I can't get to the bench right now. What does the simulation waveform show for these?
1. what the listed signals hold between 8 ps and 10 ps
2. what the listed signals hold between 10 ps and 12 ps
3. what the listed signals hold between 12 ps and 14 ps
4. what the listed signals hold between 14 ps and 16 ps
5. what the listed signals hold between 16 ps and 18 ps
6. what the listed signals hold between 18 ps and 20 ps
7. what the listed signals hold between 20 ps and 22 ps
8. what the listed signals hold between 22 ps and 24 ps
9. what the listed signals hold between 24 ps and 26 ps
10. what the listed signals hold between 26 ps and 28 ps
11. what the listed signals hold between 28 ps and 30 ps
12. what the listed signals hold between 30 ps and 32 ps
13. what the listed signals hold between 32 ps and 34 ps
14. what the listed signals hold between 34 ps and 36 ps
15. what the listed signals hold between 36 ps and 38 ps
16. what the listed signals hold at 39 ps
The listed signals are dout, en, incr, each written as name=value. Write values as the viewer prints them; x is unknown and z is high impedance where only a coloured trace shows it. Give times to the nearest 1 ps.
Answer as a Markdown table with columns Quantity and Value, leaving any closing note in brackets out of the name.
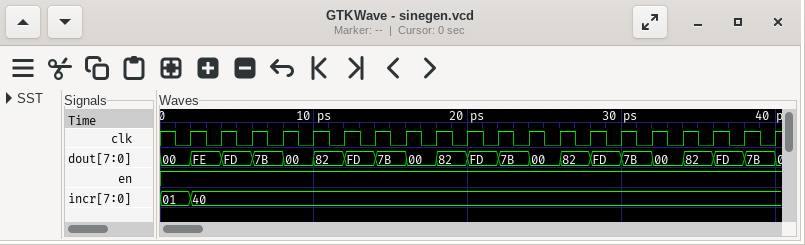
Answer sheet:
| Quantity | Value |
|---|---|
| what the listed signals hold between 8 ps and 10 ps | dout=00, en=1, incr=40 |
| what the listed signals hold between 10 ps and 12 ps | dout=82, en=1, incr=40 |
| what the listed signals hold between 12 ps and 14 ps | dout=FD, en=1, incr=40 |
| what the listed signals hold between 14 ps and 16 ps | dout=7B, en=1, incr=40 |
| what the listed signals hold between 16 ps and 18 ps | dout=00, en=1, incr=40 |
| what the listed signals hold between 18 ps and 20 ps | dout=82, en=1, incr=40 |
| what the listed signals hold between 20 ps and 22 ps | dout=FD, en=1, incr=40 |
| what the listed signals hold between 22 ps and 24 ps | dout=7B, en=1, incr=40 |
| what the listed signals hold between 24 ps and 26 ps | dout=00, en=1, incr=40 |
| what the listed signals hold between 26 ps and 28 ps | dout=82, en=1, incr=40 |
| what the listed signals hold between 28 ps and 30 ps | dout=FD, en=1, incr=40 |
| what the listed signals hold between 30 ps and 32 ps | dout=7B, en=1, incr=40 |
| what the listed signals hold between 32 ps and 34 ps | dout=00, en=1, incr=40 |
| what the listed signals hold between 34 ps and 36 ps | dout=82, en=1, incr=40 |
| what the listed signals hold between 36 ps and 38 ps | dout=FD, en=1, incr=40 |
| what the listed signals hold at 39 ps | dout=7B, en=1, incr=40 |
